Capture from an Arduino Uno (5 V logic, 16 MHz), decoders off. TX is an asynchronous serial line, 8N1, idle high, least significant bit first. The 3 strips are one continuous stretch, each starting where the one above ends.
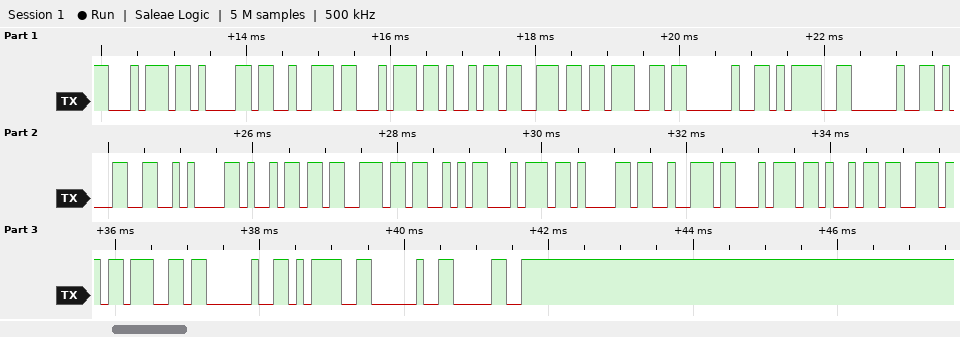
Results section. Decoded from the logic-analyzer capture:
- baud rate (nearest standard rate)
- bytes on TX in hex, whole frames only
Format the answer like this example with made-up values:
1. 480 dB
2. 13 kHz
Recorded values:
1. 9600 baud
2. 74 61 72 74 69 6E 67 20 3D 20 31 0A 69 73 53 74 61 72 74 69 6E 67 20 3D 20 30
